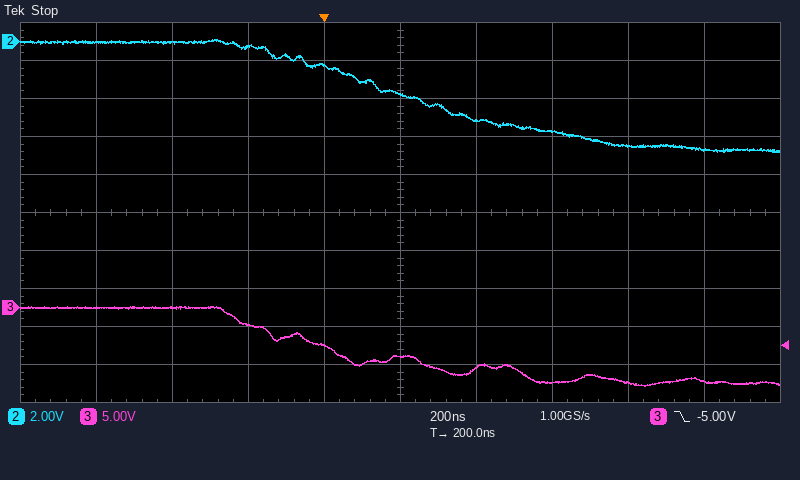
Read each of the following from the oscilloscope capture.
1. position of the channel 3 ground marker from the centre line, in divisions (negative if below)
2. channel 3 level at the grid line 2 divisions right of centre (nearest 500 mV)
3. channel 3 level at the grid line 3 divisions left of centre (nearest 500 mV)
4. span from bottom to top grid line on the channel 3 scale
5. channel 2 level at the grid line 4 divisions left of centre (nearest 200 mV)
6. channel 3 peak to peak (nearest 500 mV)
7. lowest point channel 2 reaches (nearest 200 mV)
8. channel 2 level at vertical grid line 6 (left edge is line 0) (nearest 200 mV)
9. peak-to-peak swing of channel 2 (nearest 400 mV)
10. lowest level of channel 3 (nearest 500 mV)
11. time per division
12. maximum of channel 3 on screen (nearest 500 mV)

-2.5 div
-10.0 V
0.0 V
50 V
0.0 V
10.5 V
-5.8 V
-4.2 V
6.0 V
-10.5 V
200 ns
0.0 V
